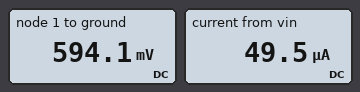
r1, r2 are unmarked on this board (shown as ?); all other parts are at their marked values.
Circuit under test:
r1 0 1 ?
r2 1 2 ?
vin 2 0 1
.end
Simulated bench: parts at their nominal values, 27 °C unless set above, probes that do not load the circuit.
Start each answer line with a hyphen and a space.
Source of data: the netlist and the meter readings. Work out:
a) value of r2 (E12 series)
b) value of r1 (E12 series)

- 8.2 kΩ
- 12 kΩ
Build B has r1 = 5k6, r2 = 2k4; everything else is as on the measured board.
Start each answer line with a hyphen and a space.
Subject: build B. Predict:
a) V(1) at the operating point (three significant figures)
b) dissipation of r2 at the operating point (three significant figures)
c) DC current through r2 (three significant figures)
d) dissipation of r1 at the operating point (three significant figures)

- 700 mV
- 37.5 µW
- 125 µA
- 87.5 µW
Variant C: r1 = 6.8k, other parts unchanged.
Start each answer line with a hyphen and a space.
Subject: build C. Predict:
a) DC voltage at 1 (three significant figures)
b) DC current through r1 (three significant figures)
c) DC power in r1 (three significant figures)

- 453 mV
- 66.7 µA
- 30.2 µW
